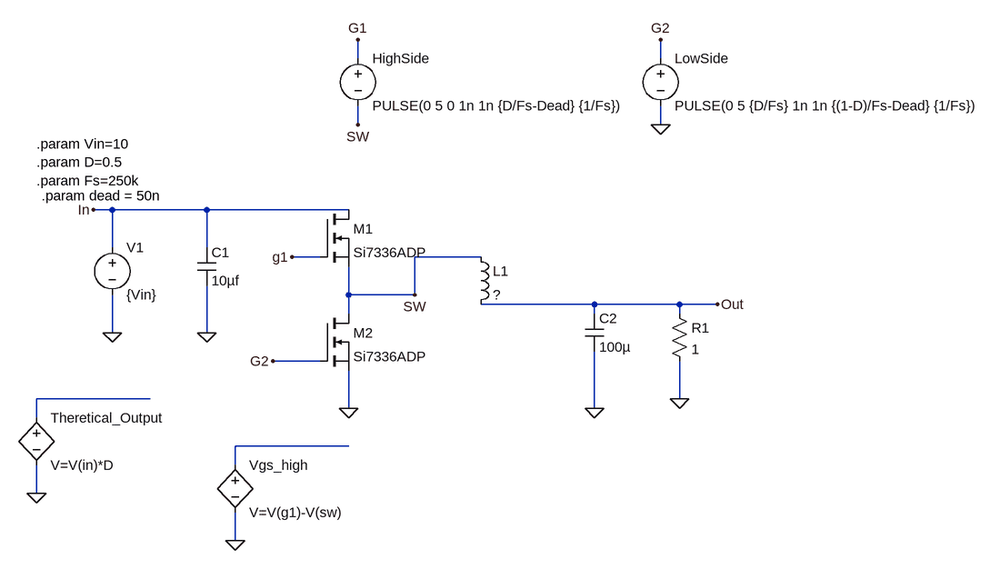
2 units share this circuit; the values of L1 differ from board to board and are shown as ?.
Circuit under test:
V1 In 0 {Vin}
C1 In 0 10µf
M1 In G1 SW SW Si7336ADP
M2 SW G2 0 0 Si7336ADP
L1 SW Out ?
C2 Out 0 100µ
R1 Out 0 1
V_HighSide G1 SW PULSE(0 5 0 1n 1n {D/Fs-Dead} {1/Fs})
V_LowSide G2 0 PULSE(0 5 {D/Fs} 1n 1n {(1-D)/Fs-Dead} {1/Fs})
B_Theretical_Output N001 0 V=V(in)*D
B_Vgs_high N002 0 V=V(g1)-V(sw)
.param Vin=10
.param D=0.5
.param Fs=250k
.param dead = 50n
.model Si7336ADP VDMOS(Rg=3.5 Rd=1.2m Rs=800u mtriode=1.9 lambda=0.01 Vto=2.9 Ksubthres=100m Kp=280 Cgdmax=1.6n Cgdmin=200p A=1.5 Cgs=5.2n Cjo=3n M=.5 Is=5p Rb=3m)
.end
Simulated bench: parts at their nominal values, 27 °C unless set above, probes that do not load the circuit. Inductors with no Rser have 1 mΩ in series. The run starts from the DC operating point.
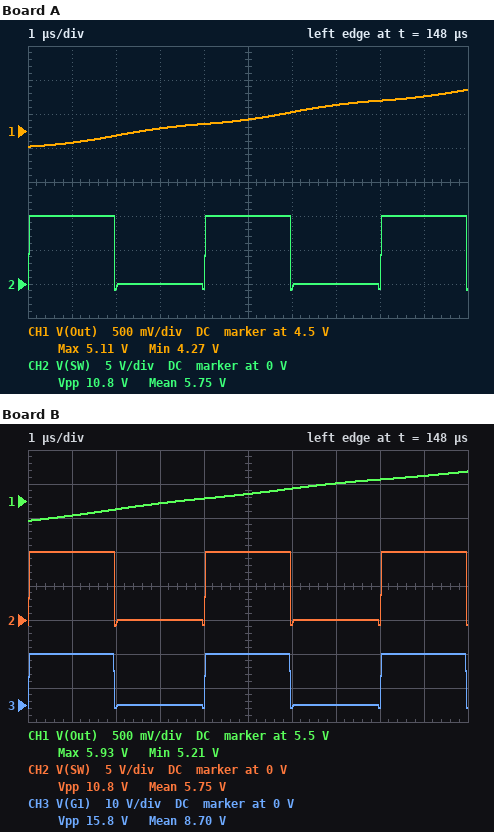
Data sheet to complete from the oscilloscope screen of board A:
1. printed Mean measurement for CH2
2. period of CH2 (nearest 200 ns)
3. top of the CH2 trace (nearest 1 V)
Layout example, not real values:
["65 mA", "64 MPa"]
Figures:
["5.75 V", "4.0 µs", "10 V"]
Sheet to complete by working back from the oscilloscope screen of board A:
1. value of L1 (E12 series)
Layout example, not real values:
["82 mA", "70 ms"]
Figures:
["1.2 µH"]
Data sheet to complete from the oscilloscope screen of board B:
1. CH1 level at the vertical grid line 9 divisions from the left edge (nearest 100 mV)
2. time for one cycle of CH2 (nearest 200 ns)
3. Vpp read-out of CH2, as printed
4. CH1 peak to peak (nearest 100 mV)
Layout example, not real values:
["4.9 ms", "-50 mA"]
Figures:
["5.9 V", "4.0 µs", "10.8 V", "700 mV"]
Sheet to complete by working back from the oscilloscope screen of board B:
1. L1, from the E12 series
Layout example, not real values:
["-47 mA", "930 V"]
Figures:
["3.3 µH"]
